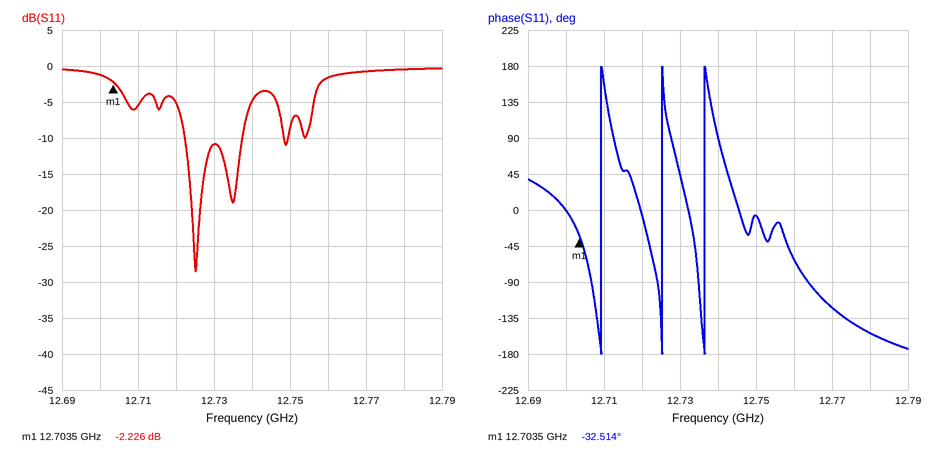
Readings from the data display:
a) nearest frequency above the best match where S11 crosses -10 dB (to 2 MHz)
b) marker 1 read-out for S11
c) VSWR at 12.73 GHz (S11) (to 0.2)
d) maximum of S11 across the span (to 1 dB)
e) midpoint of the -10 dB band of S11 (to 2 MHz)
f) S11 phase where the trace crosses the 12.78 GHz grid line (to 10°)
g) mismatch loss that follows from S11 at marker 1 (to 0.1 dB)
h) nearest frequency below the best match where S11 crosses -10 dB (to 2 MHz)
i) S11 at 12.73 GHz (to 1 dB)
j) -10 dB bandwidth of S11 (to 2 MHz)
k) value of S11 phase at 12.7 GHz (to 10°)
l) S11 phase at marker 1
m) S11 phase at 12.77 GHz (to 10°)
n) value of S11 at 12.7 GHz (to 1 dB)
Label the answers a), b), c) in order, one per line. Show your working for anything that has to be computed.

a) 12.738 GHz
b) -2.226 dB
c) |Γ| = 10^(-11/20) = 0.2818; VSWR = (1 + 0.2818)/(1 − 0.2818) ≈ 1.8
d) 0 dB
e) 12.730 GHz
f) -150°
g) −10 log10(1 − 10^(-2.226/10)) ≈ 4.0 dB
h) 12.722 GHz
i) -11 dB
j) 12.738 GHz − 12.722 GHz = 16 MHz
k) 0°
l) -32.514°
m) -120°
n) -1 dB
